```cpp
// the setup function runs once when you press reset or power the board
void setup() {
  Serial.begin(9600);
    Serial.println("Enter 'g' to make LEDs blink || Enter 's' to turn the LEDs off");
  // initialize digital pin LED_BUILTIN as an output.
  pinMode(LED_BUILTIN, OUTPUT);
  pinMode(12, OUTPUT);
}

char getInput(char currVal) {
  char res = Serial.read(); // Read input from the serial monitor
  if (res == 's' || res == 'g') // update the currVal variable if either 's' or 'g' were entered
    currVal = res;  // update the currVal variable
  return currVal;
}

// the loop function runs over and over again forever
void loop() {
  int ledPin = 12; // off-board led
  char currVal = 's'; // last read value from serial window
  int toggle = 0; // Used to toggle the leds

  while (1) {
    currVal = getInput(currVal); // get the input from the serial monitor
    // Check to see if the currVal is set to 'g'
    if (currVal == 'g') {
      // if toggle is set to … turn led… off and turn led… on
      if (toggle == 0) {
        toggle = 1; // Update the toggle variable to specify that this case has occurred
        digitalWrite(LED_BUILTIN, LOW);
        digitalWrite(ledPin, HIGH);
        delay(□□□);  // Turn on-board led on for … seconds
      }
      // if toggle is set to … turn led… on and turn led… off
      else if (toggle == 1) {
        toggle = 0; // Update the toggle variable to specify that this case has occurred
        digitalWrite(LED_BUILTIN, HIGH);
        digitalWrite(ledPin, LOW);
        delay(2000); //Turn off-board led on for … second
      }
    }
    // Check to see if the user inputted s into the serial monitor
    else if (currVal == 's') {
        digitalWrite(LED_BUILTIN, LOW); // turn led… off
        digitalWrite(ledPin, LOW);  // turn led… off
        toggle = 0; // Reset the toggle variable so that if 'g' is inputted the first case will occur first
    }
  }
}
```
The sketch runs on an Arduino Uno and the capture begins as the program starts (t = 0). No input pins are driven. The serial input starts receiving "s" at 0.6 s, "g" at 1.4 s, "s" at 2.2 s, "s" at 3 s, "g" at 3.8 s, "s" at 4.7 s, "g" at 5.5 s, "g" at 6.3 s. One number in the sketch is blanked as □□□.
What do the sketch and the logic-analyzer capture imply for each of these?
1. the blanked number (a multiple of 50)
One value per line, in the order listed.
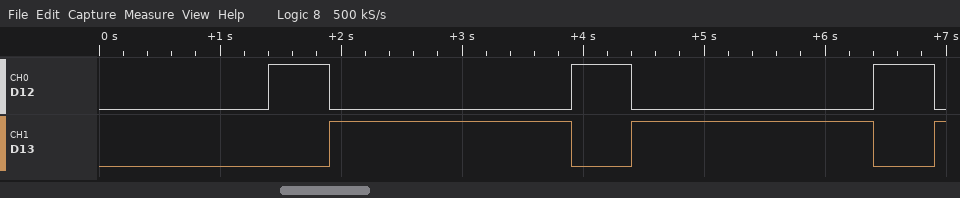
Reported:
500
